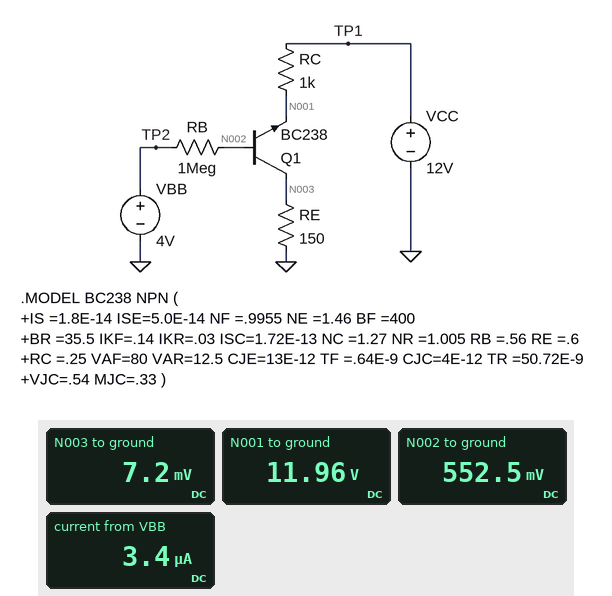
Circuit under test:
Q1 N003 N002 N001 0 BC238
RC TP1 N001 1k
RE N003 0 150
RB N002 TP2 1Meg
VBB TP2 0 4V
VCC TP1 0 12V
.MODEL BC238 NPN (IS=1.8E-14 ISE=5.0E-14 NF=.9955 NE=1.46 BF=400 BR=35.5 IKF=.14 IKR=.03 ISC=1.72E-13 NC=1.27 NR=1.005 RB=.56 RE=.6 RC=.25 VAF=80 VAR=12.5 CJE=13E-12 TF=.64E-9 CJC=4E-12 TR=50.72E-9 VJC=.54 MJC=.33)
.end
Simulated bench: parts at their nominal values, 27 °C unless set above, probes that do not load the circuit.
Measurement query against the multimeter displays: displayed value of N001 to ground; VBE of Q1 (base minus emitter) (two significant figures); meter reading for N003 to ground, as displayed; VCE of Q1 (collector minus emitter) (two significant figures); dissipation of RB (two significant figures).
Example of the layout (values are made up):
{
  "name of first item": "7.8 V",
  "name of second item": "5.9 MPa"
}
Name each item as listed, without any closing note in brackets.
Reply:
{
  "displayed value of N001 to ground": "11.96 V",
  "VBE of Q1 (base minus emitter)": "-11 V",
  "meter reading for N003 to ground, as displayed": "7.2 mV",
  "VCE of Q1 (collector minus emitter)": "-12 V",
  "dissipation of RB": "12 µW"
}
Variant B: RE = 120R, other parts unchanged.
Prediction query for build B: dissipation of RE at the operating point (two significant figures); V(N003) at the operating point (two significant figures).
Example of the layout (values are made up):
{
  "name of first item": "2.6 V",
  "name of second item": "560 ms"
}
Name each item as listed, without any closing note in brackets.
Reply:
{
  "dissipation of RE at the operating point": "270 nW",
  "V(N003) at the operating point": "5.7 mV"
}
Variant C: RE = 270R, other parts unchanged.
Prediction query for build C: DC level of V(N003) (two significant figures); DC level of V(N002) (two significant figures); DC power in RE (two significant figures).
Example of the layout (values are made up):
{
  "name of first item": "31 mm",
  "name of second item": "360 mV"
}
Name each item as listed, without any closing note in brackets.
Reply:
{
  "DC level of V(N003)": "13 mV",
  "DC level of V(N002)": "560 mV",
  "DC power in RE": "610 nW"
}
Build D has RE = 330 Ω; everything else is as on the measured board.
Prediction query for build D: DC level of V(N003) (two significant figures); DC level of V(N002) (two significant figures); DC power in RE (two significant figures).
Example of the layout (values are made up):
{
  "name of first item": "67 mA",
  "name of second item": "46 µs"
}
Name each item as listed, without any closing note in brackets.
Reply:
{
  "DC level of V(N003)": "16 mV",
  "DC level of V(N002)": "560 mV",
  "DC power in RE": "750 nW"
}
